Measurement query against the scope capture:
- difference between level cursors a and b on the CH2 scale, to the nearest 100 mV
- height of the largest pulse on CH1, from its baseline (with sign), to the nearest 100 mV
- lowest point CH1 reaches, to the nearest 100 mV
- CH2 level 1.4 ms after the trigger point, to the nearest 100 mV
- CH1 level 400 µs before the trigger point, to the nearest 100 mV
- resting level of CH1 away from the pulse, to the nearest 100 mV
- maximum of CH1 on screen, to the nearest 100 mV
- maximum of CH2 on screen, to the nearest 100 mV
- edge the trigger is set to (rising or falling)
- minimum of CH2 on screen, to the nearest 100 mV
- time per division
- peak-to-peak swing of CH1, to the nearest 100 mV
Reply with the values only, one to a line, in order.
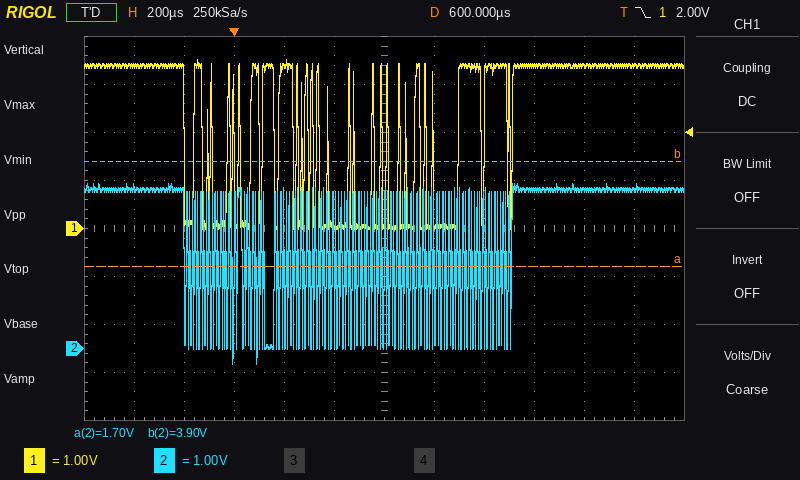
2.2 V
-3.4 V
0.0 V
3.3 V
3.4 V
3.4 V
3.5 V
3.4 V
falling
-300 mV
200 µs
3.5 V
